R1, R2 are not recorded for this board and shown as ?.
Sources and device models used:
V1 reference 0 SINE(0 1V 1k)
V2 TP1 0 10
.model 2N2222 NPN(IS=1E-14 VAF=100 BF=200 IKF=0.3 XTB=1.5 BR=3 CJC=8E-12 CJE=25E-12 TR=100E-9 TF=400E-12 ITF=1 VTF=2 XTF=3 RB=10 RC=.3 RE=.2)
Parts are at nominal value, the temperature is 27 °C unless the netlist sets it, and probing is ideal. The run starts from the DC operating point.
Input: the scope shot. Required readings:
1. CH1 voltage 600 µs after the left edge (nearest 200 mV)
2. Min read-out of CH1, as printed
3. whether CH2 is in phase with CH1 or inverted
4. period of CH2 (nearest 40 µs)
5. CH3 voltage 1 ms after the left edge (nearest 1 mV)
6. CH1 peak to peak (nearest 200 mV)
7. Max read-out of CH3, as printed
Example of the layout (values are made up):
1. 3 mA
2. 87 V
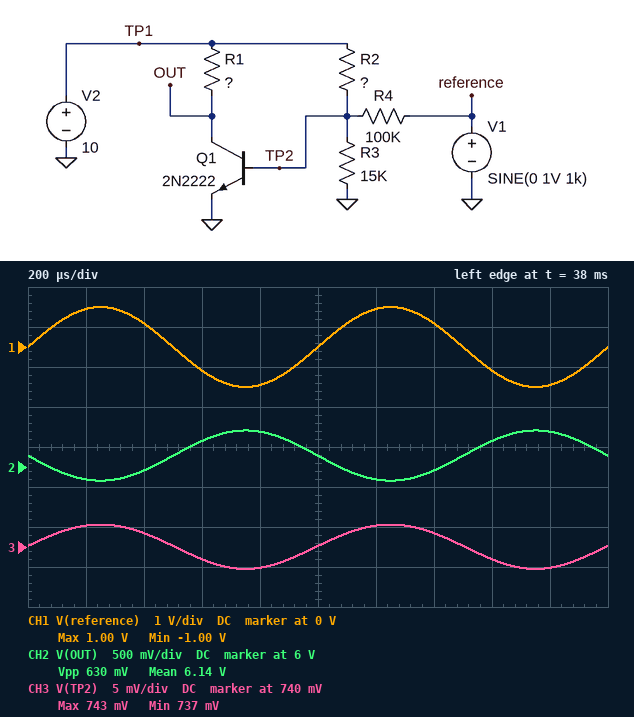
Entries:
1. -600 mV
2. -1.00 V
3. inverted
4. 1.00 ms
5. 740 mV
6. 2.0 V
7. 743 mV
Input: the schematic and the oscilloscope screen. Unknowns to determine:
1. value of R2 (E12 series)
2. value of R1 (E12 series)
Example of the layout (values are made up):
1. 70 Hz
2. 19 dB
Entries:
1. 56 kΩ
2. 180 Ω
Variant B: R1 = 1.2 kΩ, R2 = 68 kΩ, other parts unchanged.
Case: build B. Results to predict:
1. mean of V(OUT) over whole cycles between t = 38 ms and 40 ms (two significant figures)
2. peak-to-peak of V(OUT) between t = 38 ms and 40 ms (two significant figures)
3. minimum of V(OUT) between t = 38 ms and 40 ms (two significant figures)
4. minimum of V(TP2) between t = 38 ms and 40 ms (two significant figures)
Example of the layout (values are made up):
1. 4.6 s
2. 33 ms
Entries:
1. 120 mV
2. 13 mV
3. 110 mV
4. 710 mV
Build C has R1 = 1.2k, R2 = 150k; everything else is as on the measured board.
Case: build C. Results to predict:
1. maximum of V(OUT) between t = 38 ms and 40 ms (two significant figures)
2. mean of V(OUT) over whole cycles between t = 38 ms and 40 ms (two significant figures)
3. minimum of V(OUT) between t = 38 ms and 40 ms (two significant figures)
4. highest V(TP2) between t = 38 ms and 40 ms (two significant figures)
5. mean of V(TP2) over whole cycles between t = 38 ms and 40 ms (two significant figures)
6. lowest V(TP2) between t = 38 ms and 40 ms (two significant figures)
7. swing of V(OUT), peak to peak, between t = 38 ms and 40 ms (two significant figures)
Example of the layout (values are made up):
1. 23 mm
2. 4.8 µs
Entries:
1. 9.2 V
2. 7.3 V
3. 5.3 V
4. 690 mV
5. 670 mV
6. 640 mV
7. 3.9 V
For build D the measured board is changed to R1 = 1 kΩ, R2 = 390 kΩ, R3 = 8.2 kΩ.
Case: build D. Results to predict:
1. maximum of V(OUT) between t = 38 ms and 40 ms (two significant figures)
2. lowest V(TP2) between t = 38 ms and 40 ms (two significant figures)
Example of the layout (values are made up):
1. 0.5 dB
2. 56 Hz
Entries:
1. 10 V
2. 120 mV
